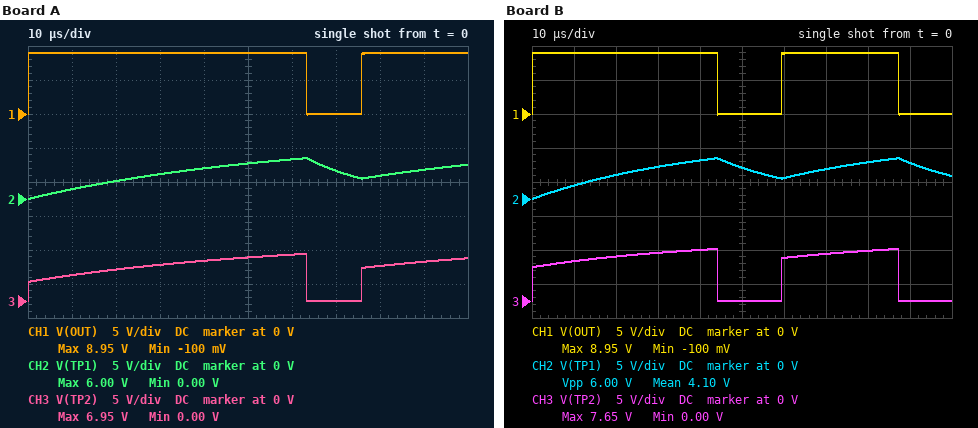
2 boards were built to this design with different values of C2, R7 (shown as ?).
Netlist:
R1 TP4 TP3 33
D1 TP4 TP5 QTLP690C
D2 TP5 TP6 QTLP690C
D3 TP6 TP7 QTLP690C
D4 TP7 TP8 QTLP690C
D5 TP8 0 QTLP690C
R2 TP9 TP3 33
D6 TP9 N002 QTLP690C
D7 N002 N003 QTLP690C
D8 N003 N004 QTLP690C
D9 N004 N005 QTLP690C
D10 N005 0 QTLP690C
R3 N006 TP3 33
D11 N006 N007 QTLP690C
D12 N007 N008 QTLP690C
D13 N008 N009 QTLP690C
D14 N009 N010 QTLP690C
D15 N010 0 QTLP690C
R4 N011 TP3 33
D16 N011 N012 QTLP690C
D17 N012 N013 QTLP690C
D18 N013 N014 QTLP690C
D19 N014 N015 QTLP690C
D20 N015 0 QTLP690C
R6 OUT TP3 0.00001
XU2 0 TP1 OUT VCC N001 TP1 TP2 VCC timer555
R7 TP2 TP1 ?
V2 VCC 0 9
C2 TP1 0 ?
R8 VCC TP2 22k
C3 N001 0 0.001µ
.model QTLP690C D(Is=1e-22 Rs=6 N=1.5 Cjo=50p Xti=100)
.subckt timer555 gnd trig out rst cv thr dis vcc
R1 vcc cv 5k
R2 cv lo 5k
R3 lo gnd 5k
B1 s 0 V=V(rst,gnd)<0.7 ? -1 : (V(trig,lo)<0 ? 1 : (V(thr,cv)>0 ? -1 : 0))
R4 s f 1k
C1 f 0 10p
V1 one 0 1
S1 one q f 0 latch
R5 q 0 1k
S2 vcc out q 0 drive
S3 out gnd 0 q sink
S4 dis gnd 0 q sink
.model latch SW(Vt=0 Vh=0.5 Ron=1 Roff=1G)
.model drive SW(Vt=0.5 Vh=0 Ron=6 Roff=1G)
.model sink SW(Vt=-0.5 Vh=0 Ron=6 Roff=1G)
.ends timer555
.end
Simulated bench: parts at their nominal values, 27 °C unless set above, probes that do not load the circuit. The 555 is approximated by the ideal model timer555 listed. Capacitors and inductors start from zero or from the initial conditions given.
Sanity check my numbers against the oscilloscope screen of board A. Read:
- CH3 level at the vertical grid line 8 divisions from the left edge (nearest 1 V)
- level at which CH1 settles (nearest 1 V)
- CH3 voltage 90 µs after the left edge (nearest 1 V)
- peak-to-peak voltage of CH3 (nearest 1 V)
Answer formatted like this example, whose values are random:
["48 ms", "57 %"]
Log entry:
["5 V", "9 V", "6 V", "7 V"]
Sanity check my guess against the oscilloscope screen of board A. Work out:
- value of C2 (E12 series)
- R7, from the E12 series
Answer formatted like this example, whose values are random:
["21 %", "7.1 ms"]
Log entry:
["1.8 nF", "10 kΩ"]
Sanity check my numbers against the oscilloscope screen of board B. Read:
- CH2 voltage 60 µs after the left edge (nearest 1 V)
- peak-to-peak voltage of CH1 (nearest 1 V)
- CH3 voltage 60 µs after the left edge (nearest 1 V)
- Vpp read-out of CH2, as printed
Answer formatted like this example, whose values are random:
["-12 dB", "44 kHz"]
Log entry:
["3 V", "9 V", "6 V", "6.00 V"]
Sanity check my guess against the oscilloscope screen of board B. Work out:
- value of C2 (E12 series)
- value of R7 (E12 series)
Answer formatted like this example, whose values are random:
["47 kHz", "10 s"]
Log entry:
["820 pF", "27 kΩ"]
